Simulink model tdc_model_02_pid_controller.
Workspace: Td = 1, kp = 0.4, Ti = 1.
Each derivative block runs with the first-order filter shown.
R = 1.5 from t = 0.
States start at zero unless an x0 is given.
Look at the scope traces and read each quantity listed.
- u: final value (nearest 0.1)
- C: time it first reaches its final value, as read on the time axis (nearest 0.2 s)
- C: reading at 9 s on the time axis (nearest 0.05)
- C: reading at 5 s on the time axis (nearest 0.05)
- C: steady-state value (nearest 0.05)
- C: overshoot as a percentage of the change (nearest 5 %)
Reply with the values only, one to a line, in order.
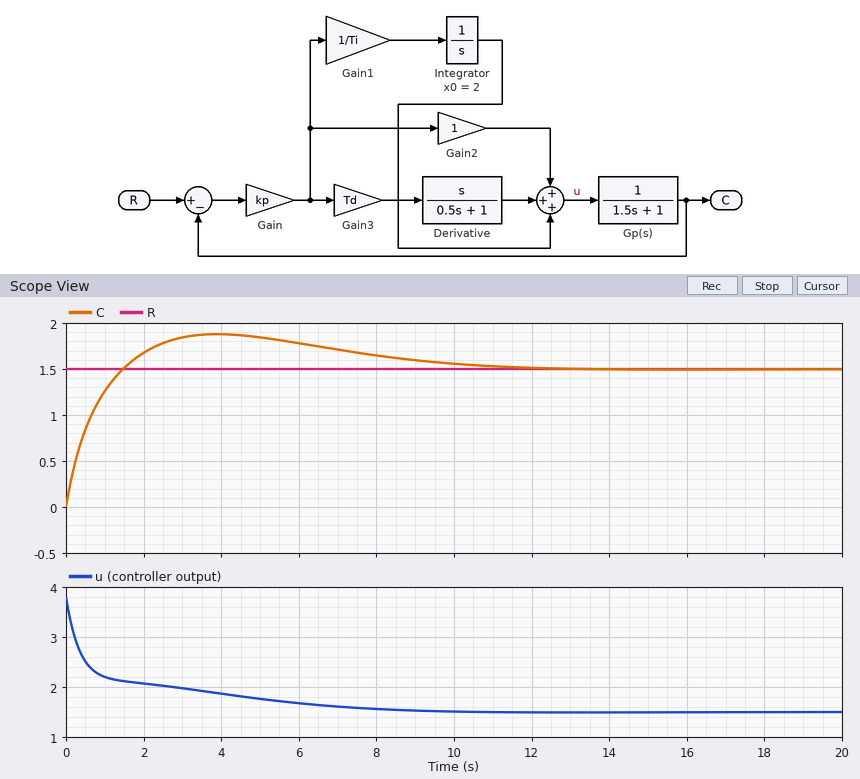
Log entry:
1.5
1.4 s
1.60
1.85
1.50
25 %
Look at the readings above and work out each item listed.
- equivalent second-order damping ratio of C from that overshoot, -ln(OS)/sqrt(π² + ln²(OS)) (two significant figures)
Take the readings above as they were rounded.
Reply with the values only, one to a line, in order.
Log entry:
0.40
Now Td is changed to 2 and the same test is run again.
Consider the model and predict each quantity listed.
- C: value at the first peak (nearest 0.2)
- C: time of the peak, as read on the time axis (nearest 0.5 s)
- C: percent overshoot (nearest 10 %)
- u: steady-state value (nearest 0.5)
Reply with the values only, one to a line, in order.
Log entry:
1.8
4.5 s
20 %
1.5
